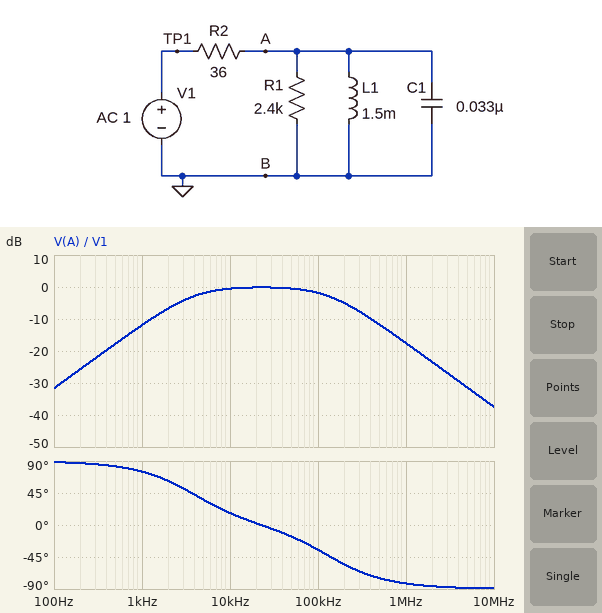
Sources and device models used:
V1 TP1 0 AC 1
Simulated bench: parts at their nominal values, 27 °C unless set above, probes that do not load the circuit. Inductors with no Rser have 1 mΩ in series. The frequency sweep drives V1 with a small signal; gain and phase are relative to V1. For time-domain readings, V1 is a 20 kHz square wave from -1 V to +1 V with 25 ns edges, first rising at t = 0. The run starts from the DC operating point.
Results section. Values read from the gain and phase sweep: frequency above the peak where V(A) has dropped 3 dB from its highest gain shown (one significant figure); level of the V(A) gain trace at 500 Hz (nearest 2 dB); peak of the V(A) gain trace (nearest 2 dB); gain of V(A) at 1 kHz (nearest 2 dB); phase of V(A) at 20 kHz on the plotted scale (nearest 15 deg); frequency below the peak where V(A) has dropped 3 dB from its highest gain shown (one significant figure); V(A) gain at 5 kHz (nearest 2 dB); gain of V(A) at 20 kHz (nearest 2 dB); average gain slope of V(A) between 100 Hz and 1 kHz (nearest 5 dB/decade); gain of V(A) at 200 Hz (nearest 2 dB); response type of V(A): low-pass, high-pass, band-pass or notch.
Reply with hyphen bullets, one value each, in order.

- 100 kHz
- -18 dB
- 0 dB
- -12 dB
- 0 deg
- 4 kHz
- -2 dB
- 0 dB
- 20 dB/decade
- -26 dB
- band-pass
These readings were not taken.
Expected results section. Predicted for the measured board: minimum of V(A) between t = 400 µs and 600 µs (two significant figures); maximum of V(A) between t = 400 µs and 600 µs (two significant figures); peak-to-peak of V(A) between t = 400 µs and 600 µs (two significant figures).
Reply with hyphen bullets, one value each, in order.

- -1.2 V
- 1.2 V
- 2.3 V
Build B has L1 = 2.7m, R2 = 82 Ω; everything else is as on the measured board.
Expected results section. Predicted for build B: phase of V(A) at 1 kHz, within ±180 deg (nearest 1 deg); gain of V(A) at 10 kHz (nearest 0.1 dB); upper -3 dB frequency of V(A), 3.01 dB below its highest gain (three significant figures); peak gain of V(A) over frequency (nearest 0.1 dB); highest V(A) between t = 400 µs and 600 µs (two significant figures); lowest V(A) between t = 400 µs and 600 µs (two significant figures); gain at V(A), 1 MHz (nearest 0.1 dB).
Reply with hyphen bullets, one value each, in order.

- 78 deg
- -0.7 dB
- 65.2 kHz
- -0.3 dB
- 1.1 V
- -1.1 V
- -24.6 dB
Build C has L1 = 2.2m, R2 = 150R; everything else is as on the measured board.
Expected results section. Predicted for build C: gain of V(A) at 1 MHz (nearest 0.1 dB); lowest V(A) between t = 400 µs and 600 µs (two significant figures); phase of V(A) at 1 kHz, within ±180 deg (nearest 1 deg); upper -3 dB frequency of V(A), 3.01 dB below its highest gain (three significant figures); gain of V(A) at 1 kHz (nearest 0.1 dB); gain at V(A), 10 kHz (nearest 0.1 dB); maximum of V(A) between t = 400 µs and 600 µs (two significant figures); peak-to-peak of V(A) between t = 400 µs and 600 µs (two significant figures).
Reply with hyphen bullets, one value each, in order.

- -29.9 dB
- -1.1 V
- 84 deg
- 42.4 kHz
- -20.7 dB
- -2.4 dB
- 1.1 V
- 2.3 V
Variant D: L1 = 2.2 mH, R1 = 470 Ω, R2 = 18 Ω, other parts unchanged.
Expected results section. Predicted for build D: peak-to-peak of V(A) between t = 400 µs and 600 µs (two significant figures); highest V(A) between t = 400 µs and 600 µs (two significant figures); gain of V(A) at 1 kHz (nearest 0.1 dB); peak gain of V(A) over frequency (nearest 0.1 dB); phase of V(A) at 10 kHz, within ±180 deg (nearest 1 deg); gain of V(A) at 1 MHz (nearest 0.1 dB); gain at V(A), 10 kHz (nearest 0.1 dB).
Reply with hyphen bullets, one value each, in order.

- 2.1 V
- 1.1 V
- -4.4 dB
- -0.3 dB
- 5 deg
- -11.8 dB
- -0.4 dB
